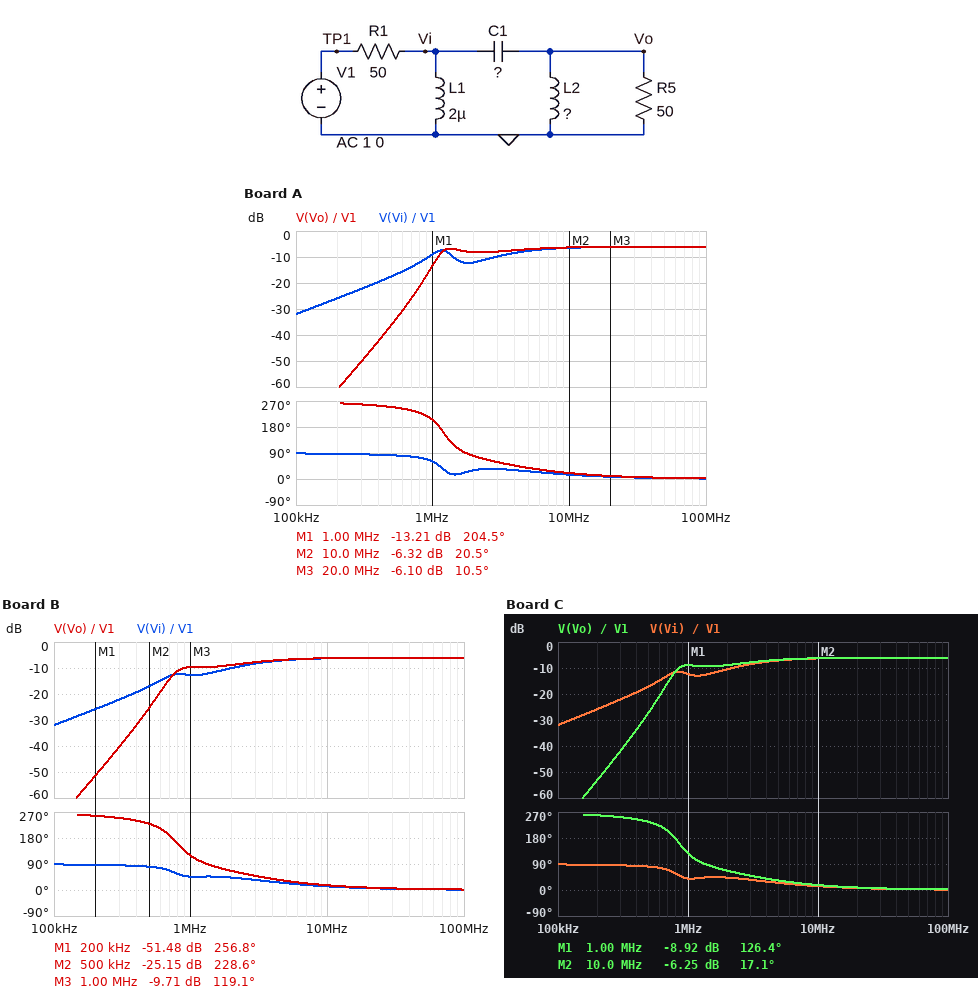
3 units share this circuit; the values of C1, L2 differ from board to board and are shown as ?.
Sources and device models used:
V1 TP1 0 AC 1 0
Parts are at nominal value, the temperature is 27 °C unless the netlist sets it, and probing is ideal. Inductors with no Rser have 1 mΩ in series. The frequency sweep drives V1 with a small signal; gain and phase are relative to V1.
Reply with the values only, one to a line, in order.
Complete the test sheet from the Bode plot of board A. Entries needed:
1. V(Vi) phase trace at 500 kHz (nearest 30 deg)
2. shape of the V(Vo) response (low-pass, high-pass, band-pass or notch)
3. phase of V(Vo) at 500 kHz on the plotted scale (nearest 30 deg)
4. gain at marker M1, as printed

90 deg
high-pass
240 deg
-13.21 dB
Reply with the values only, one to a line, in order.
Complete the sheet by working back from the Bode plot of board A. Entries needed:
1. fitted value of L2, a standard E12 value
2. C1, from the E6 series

3.3 µH
3.3 nF
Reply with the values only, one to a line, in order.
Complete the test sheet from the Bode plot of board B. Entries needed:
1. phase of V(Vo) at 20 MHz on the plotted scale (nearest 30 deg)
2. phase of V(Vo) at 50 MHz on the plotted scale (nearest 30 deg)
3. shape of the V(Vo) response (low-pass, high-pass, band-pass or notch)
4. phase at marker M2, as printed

0 deg
0 deg
high-pass
228.6 deg
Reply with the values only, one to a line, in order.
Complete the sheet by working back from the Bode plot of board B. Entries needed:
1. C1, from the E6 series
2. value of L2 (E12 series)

4.7 nF
6.8 µH
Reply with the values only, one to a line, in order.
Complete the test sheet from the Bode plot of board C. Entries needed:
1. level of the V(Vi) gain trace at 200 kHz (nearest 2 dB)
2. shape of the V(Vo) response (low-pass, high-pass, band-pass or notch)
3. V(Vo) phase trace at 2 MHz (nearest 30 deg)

-26 dB
high-pass
60 deg
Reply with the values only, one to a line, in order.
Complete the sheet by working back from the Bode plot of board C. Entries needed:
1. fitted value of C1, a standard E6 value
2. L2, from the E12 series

4.7 nF
5.6 µH
